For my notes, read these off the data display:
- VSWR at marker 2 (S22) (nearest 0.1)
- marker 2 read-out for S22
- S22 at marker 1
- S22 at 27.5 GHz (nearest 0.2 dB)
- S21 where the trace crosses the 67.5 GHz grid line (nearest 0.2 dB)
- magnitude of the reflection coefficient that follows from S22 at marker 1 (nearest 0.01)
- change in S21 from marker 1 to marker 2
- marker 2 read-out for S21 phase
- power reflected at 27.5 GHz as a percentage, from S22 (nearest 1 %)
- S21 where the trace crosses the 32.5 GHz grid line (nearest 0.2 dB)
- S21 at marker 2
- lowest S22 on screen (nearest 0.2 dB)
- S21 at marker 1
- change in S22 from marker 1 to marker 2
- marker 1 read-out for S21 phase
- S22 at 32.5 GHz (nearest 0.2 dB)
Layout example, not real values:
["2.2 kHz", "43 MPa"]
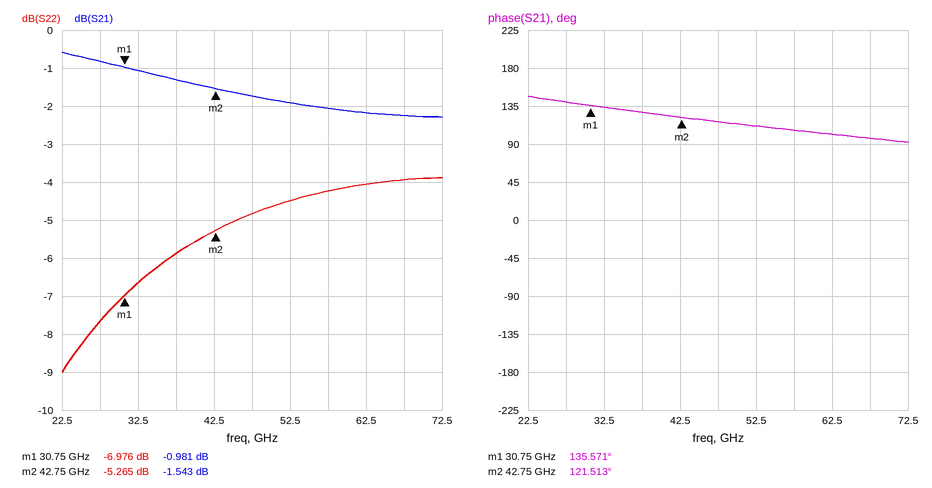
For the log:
["3.4", "-5.265 dB", "-6.976 dB", "-7.6 dB", "-2.2 dB", "0.45", "-0.562 dB", "121.513°", "17 %", "-1.0 dB", "-1.543 dB", "-9.0 dB", "-0.981 dB", "1.711 dB", "135.571°", "-6.6 dB"]
